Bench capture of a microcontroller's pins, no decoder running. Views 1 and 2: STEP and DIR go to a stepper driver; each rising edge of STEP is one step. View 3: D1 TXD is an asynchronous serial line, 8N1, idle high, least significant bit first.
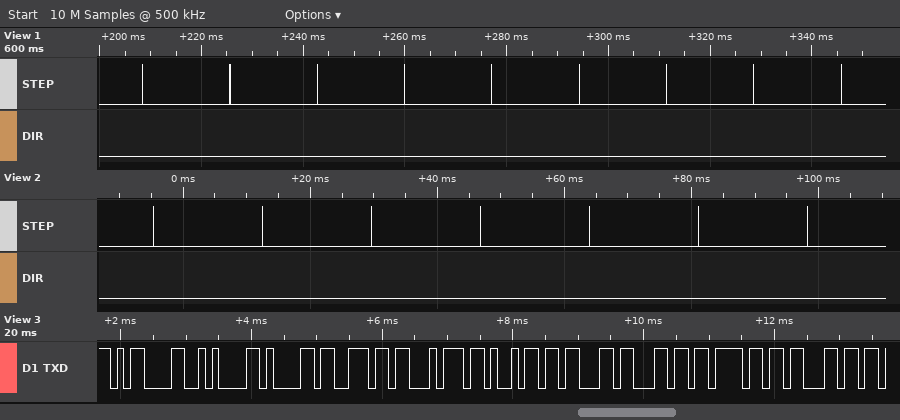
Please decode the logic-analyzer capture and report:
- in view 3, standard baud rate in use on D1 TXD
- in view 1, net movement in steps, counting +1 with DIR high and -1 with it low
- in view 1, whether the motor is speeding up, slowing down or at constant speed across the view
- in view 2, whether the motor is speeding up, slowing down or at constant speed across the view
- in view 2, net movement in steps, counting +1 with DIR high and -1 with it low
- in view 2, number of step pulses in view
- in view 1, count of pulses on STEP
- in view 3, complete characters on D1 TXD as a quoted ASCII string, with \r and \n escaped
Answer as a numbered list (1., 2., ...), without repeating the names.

1. 9600 baud
2. -9
3. constant speed
4. constant speed
5. -7
6. 7
7. 9
8. "\r\nanticloc"
